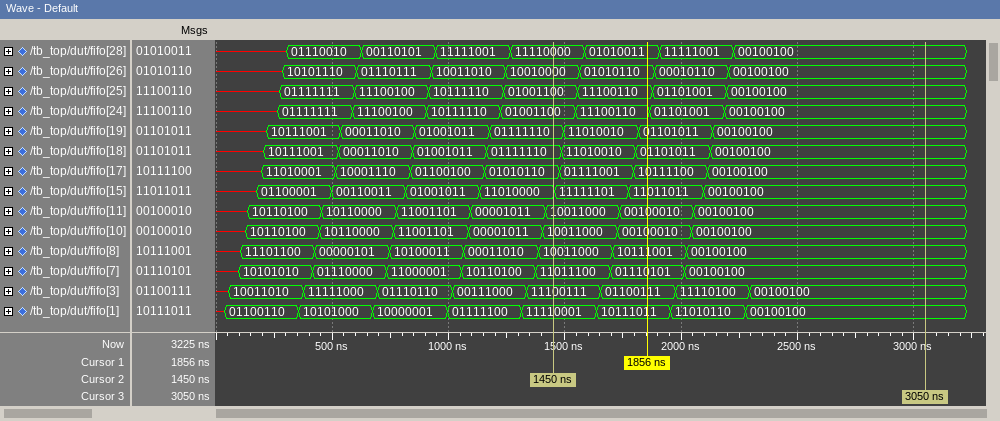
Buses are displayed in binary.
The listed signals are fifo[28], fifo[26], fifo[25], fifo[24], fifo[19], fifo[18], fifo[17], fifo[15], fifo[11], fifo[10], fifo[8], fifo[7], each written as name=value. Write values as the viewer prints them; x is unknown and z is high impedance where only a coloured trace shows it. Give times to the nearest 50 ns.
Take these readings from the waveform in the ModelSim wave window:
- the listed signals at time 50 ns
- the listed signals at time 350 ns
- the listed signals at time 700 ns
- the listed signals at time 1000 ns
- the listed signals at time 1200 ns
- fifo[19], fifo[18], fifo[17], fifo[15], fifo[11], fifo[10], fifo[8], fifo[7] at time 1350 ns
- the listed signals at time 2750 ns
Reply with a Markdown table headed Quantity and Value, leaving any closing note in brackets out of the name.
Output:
| Quantity | Value |
|---|---|
| the listed signals at time 50 ns | fifo[28]=x, fifo[26]=x, fifo[25]=x, fifo[24]=x, fifo[19]=x, fifo[18]=x, fifo[17]=x, fifo[15]=x, fifo[11]=x, fifo[10]=x, fifo[8]=x, fifo[7]=x |
| the listed signals at time 350 ns | fifo[28]=01110010, fifo[26]=10101110, fifo[25]=01111111, fifo[24]=01111111, fifo[19]=10111001, fifo[18]=10111001, fifo[17]=11010001, fifo[15]=01100001, fifo[11]=10110100, fifo[10]=10110100, fifo[8]=11101100, fifo[7]=10101010 |
| the listed signals at time 700 ns | fifo[28]=00110101, fifo[26]=01110111, fifo[25]=11100100, fifo[24]=11100100, fifo[19]=00011010, fifo[18]=00011010, fifo[17]=10001110, fifo[15]=00110011, fifo[11]=10110000, fifo[10]=10110000, fifo[8]=00000101, fifo[7]=01110000 |
| the listed signals at time 1000 ns | fifo[28]=11111001, fifo[26]=10011010, fifo[25]=10111110, fifo[24]=10111110, fifo[19]=01001011, fifo[18]=01001011, fifo[17]=01100100, fifo[15]=01001011, fifo[11]=11001101, fifo[10]=11001101, fifo[8]=10100011, fifo[7]=11000001 |
| the listed signals at time 1200 ns | fifo[28]=11111001, fifo[26]=10011010, fifo[25]=10111110, fifo[24]=10111110, fifo[19]=01111110, fifo[18]=01111110, fifo[17]=01010110, fifo[15]=11010000, fifo[11]=00001011, fifo[10]=00001011, fifo[8]=00011010, fifo[7]=10110100 |
| fifo[19], fifo[18], fifo[17], fifo[15], fifo[11], fifo[10], fifo[8], fifo[7] at time 1350 ns | fifo[19]=01111110, fifo[18]=01111110, fifo[17]=01010110, fifo[15]=11010000, fifo[11]=00001011, fifo[10]=00001011, fifo[8]=00011010, fifo[7]=10110100 |
| the listed signals at time 2750 ns | fifo[28]=00100100, fifo[26]=00100100, fifo[25]=00100100, fifo[24]=00100100, fifo[19]=00100100, fifo[18]=00100100, fifo[17]=00100100, fifo[15]=00100100, fifo[11]=00100100, fifo[10]=00100100, fifo[8]=00100100, fifo[7]=00100100 |
